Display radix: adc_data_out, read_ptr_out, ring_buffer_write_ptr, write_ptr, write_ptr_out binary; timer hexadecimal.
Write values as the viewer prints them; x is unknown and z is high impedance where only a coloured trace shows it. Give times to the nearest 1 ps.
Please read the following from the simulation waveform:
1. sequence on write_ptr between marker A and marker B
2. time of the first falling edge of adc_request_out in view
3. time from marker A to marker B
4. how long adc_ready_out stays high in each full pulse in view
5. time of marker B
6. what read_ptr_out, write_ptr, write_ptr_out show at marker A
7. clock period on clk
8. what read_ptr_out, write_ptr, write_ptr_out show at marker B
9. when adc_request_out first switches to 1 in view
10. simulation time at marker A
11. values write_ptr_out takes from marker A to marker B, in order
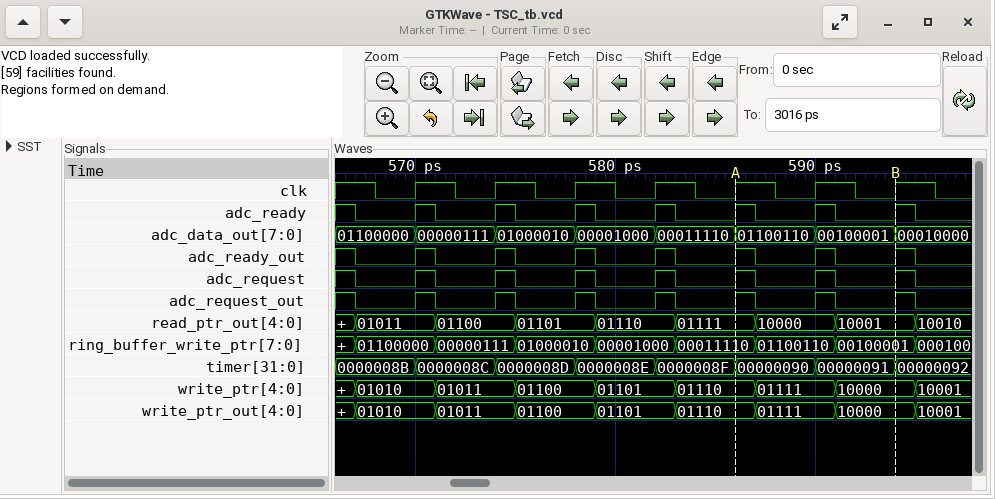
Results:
01110, 01111, 10000
567 ps
8 ps
1 ps, 1 ps, 1 ps, 1 ps, 1 ps, 1 ps, 1 ps
594 ps
read_ptr_out=01111, write_ptr=01110, write_ptr_out=01110
4 ps
read_ptr_out=10001, write_ptr=10000, write_ptr_out=10000
570 ps
586 ps
01110, 01111, 10000
